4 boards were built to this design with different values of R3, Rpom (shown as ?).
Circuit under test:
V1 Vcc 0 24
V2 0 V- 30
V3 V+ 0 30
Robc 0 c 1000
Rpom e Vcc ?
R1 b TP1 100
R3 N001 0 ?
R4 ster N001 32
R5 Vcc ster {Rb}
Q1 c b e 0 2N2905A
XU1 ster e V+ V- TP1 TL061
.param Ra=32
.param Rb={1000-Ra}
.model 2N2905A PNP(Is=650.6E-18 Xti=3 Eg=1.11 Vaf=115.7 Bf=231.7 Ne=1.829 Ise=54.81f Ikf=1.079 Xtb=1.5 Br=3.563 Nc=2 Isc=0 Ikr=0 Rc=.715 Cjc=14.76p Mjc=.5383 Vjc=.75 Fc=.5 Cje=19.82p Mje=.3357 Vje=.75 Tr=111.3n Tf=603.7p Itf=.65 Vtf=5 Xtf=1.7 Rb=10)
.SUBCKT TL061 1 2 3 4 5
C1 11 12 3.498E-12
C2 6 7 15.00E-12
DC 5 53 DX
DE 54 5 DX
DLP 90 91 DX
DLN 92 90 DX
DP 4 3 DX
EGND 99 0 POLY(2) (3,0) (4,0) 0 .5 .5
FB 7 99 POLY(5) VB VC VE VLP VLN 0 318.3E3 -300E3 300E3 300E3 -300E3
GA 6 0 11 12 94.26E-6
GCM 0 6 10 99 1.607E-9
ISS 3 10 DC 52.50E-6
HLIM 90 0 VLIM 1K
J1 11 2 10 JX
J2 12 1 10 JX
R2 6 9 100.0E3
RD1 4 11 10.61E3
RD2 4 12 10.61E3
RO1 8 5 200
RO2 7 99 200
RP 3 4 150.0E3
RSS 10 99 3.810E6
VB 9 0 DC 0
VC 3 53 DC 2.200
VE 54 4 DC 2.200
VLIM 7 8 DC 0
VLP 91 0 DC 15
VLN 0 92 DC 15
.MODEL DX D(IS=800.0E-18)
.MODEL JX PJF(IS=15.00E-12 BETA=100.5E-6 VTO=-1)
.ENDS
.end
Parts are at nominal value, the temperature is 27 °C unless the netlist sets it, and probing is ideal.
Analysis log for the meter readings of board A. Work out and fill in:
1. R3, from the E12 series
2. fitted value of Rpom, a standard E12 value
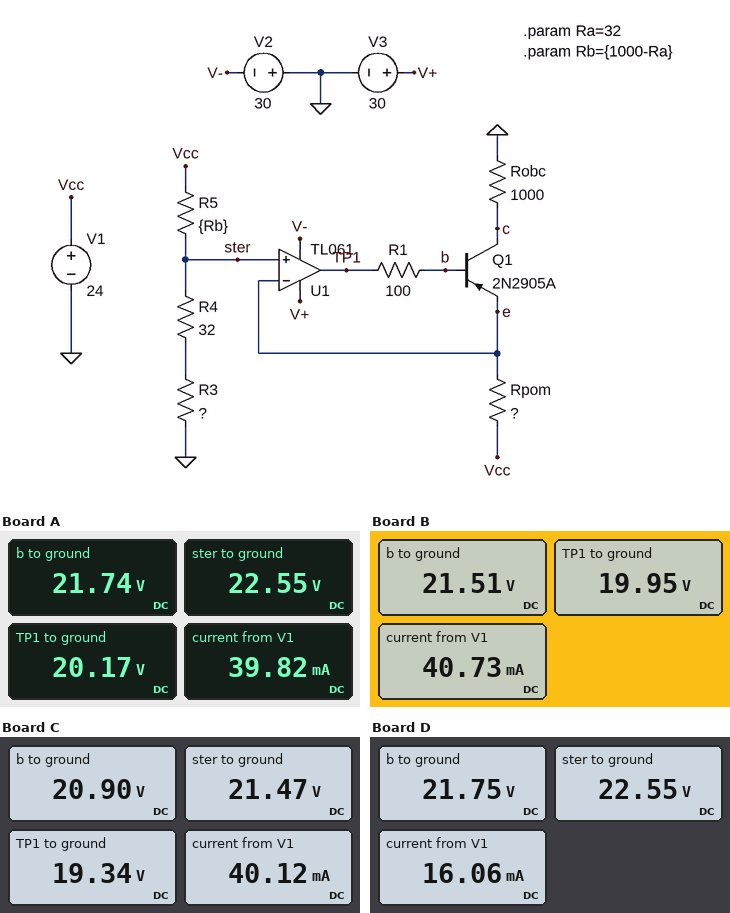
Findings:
15 kΩ
33 Ω
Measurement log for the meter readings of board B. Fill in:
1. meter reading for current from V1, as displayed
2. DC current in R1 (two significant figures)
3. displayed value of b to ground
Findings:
40.73 mA
16 mA
21.51 V
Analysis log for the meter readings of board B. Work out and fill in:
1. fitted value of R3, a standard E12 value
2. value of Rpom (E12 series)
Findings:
8.2 kΩ
39 Ω
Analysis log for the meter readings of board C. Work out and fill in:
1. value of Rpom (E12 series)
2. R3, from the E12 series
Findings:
56 Ω
8.2 kΩ
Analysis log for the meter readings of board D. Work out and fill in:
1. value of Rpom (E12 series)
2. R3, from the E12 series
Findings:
100 Ω
15 kΩ
